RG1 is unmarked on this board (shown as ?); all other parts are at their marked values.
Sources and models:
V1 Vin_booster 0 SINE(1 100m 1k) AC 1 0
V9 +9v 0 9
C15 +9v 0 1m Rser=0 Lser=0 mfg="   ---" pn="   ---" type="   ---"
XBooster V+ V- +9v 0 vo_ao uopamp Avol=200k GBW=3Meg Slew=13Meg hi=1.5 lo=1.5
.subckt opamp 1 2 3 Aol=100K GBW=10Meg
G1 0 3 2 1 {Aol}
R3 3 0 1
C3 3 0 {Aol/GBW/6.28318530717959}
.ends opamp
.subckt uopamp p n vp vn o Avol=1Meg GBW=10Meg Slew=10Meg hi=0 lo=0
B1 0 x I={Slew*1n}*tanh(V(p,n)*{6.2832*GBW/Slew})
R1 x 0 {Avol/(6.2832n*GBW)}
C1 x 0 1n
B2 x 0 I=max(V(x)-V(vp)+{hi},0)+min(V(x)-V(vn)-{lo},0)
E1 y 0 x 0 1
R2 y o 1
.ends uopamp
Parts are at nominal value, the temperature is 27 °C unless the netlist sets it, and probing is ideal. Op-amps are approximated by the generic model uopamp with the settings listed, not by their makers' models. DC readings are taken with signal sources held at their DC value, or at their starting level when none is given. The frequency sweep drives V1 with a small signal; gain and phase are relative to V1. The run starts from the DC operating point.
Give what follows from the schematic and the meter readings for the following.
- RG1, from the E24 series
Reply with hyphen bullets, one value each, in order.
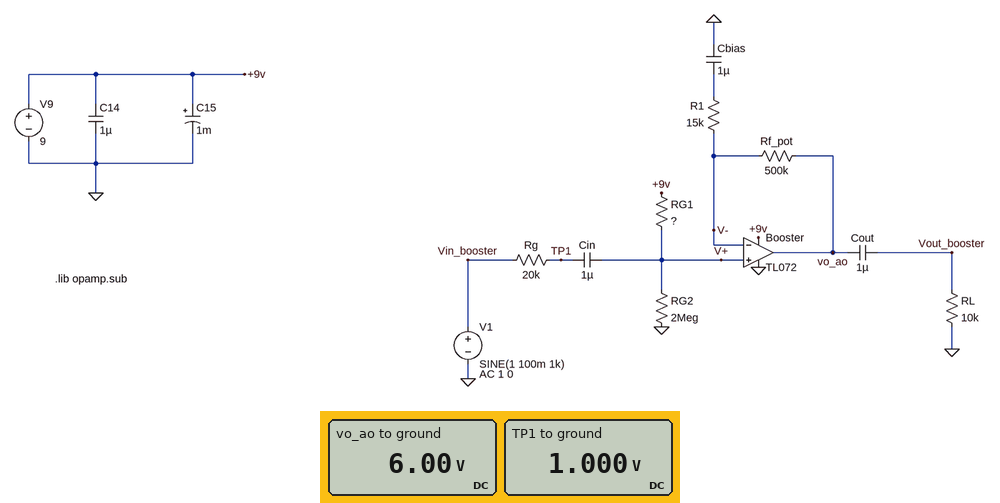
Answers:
- 1 MΩ
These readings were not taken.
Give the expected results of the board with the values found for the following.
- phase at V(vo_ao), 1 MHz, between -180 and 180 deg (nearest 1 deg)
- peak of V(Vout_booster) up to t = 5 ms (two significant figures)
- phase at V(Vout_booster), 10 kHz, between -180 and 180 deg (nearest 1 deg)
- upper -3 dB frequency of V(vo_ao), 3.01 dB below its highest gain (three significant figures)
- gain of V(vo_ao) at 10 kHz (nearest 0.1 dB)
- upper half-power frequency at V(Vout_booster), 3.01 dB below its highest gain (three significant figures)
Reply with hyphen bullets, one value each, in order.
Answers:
- -85 deg
- 1.6 V
- -6 deg
- 87.4 kHz
- 30.4 dB
- 87.4 kHz
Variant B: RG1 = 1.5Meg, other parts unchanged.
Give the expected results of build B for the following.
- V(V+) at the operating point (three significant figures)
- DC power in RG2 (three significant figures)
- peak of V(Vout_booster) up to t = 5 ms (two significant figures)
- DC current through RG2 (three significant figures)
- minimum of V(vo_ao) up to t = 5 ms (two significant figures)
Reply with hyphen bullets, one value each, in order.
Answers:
- 5.14 V
- 13.2 µW
- 2.4 V
- 2.57 µA
- 1.8 V
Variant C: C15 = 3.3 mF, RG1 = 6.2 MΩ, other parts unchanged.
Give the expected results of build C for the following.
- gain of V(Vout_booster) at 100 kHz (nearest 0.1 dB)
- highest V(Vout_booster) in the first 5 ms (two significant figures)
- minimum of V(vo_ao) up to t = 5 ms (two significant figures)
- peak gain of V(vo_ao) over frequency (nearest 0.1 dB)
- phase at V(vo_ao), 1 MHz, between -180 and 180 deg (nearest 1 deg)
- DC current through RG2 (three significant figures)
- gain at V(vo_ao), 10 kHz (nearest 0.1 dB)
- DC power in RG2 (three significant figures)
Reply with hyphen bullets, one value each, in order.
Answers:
- 27.0 dB
- 3.3 V
- 1.5 V
- 30.6 dB
- -85 deg
- 1.10 µA
- 30.5 dB
- 2.41 µW
